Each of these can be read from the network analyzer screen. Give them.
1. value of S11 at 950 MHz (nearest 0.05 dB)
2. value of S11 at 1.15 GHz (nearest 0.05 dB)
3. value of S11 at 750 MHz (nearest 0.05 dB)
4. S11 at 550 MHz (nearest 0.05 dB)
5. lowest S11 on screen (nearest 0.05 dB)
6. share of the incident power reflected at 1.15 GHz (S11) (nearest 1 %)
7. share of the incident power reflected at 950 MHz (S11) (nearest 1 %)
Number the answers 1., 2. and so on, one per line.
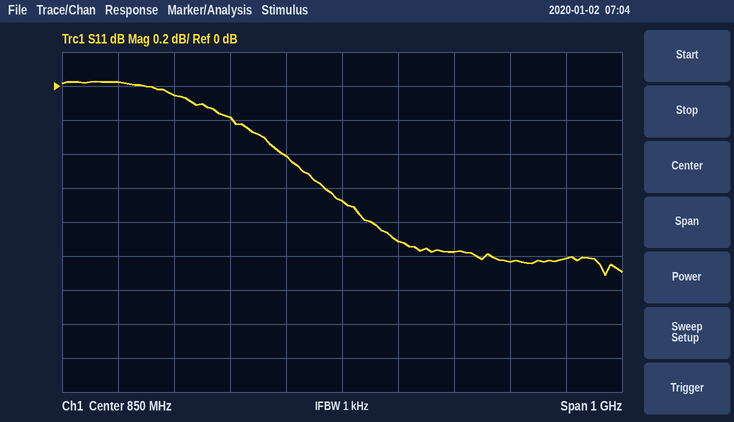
1. -0.90 dB
2. -1.05 dB
3. -0.40 dB
4. -0.05 dB
5. -1.10 dB
6. 79 %
7. 81 %
